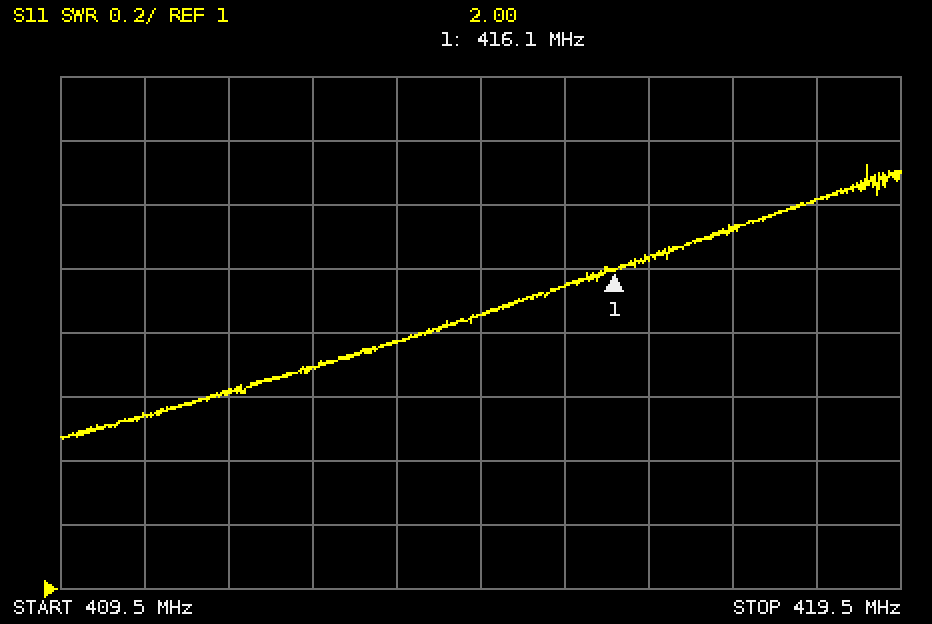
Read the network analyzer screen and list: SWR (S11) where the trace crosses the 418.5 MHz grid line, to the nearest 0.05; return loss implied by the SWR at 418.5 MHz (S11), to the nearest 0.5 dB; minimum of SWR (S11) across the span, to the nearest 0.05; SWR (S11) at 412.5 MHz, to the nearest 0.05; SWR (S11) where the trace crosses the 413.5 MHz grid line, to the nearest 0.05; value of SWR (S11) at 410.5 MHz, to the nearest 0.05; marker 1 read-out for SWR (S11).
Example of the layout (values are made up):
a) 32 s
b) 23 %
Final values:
a) 2.20
b) 8.5 dB
c) 1.45
d) 1.70
e) 1.75
f) 1.55
g) 2.00
